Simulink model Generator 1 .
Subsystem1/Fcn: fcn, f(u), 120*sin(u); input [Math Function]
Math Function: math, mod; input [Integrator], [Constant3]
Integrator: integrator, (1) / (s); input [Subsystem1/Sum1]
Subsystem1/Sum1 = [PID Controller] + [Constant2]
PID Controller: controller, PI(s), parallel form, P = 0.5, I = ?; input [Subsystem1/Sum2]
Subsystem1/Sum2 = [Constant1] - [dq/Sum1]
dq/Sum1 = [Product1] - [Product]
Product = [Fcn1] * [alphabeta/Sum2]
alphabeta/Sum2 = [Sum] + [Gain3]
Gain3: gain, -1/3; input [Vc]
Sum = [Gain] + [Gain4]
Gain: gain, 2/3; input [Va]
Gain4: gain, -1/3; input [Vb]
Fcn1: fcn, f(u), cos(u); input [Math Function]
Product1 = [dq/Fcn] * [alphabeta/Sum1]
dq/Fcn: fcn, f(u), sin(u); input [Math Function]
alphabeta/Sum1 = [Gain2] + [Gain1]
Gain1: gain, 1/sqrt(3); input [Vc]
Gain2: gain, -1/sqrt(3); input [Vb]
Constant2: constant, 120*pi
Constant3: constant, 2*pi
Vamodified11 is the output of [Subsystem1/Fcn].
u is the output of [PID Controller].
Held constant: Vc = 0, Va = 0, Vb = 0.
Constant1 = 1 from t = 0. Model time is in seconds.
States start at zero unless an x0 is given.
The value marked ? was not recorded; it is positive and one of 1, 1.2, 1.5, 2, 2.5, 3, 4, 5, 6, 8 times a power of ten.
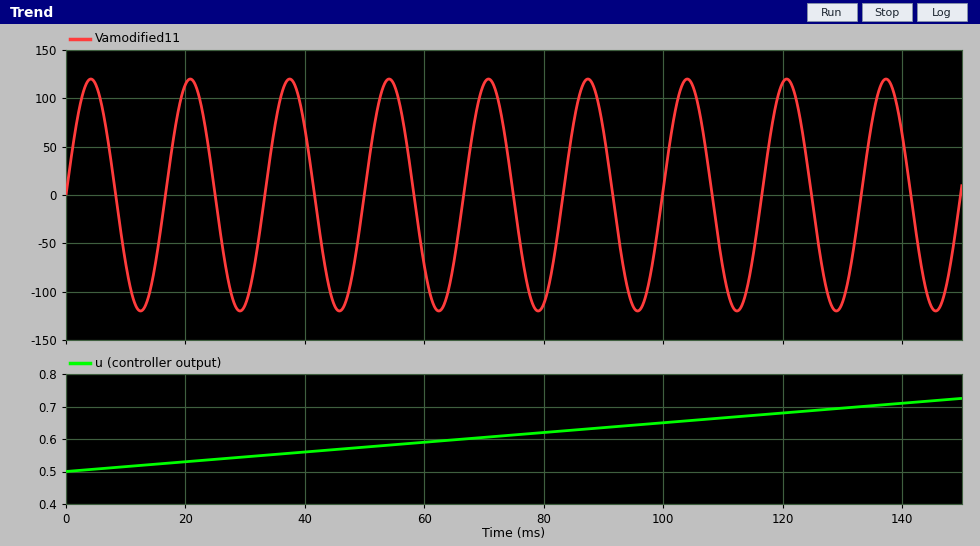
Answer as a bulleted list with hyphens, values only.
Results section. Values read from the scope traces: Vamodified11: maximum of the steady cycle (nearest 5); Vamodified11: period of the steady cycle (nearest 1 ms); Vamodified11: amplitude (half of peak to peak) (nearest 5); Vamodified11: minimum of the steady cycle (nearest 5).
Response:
- 120
- 17 ms
- 120
- -120
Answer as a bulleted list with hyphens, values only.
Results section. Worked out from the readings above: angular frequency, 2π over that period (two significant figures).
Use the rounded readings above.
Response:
- 0.37 rad/ms
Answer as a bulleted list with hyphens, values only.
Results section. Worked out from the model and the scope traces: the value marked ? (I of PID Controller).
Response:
- 1.5
